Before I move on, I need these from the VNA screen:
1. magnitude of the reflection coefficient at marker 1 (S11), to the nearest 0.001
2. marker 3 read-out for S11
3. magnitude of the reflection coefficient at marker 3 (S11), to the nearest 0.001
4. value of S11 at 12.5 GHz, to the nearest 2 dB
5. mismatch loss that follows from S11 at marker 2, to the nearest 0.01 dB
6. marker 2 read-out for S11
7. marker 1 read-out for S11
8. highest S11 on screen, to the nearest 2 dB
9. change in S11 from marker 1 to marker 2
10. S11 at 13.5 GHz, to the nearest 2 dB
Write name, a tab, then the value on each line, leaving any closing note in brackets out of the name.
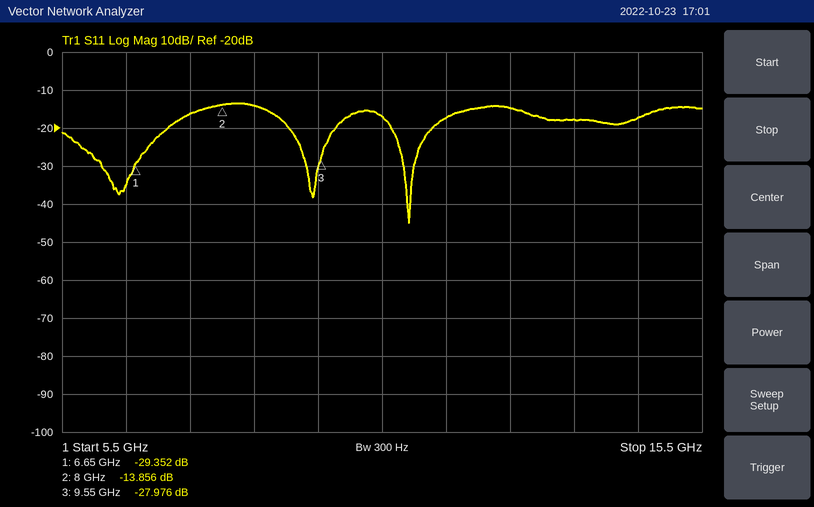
magnitude of the reflection coefficient at marker 1 (S11), to the nearest 0.001	0.034
marker 3 read-out for S11	-27.976 dB
magnitude of the reflection coefficient at marker 3 (S11), to the nearest 0.001	0.040
value of S11 at 12.5 GHz, to the nearest 2 dB	-14 dB
mismatch loss that follows from S11 at marker 2, to the nearest 0.01 dB	0.18 dB
marker 2 read-out for S11	-13.856 dB
marker 1 read-out for S11	-29.352 dB
highest S11 on screen, to the nearest 2 dB	-14 dB
change in S11 from marker 1 to marker 2	15.496 dB
S11 at 13.5 GHz, to the nearest 2 dB	-18 dB
